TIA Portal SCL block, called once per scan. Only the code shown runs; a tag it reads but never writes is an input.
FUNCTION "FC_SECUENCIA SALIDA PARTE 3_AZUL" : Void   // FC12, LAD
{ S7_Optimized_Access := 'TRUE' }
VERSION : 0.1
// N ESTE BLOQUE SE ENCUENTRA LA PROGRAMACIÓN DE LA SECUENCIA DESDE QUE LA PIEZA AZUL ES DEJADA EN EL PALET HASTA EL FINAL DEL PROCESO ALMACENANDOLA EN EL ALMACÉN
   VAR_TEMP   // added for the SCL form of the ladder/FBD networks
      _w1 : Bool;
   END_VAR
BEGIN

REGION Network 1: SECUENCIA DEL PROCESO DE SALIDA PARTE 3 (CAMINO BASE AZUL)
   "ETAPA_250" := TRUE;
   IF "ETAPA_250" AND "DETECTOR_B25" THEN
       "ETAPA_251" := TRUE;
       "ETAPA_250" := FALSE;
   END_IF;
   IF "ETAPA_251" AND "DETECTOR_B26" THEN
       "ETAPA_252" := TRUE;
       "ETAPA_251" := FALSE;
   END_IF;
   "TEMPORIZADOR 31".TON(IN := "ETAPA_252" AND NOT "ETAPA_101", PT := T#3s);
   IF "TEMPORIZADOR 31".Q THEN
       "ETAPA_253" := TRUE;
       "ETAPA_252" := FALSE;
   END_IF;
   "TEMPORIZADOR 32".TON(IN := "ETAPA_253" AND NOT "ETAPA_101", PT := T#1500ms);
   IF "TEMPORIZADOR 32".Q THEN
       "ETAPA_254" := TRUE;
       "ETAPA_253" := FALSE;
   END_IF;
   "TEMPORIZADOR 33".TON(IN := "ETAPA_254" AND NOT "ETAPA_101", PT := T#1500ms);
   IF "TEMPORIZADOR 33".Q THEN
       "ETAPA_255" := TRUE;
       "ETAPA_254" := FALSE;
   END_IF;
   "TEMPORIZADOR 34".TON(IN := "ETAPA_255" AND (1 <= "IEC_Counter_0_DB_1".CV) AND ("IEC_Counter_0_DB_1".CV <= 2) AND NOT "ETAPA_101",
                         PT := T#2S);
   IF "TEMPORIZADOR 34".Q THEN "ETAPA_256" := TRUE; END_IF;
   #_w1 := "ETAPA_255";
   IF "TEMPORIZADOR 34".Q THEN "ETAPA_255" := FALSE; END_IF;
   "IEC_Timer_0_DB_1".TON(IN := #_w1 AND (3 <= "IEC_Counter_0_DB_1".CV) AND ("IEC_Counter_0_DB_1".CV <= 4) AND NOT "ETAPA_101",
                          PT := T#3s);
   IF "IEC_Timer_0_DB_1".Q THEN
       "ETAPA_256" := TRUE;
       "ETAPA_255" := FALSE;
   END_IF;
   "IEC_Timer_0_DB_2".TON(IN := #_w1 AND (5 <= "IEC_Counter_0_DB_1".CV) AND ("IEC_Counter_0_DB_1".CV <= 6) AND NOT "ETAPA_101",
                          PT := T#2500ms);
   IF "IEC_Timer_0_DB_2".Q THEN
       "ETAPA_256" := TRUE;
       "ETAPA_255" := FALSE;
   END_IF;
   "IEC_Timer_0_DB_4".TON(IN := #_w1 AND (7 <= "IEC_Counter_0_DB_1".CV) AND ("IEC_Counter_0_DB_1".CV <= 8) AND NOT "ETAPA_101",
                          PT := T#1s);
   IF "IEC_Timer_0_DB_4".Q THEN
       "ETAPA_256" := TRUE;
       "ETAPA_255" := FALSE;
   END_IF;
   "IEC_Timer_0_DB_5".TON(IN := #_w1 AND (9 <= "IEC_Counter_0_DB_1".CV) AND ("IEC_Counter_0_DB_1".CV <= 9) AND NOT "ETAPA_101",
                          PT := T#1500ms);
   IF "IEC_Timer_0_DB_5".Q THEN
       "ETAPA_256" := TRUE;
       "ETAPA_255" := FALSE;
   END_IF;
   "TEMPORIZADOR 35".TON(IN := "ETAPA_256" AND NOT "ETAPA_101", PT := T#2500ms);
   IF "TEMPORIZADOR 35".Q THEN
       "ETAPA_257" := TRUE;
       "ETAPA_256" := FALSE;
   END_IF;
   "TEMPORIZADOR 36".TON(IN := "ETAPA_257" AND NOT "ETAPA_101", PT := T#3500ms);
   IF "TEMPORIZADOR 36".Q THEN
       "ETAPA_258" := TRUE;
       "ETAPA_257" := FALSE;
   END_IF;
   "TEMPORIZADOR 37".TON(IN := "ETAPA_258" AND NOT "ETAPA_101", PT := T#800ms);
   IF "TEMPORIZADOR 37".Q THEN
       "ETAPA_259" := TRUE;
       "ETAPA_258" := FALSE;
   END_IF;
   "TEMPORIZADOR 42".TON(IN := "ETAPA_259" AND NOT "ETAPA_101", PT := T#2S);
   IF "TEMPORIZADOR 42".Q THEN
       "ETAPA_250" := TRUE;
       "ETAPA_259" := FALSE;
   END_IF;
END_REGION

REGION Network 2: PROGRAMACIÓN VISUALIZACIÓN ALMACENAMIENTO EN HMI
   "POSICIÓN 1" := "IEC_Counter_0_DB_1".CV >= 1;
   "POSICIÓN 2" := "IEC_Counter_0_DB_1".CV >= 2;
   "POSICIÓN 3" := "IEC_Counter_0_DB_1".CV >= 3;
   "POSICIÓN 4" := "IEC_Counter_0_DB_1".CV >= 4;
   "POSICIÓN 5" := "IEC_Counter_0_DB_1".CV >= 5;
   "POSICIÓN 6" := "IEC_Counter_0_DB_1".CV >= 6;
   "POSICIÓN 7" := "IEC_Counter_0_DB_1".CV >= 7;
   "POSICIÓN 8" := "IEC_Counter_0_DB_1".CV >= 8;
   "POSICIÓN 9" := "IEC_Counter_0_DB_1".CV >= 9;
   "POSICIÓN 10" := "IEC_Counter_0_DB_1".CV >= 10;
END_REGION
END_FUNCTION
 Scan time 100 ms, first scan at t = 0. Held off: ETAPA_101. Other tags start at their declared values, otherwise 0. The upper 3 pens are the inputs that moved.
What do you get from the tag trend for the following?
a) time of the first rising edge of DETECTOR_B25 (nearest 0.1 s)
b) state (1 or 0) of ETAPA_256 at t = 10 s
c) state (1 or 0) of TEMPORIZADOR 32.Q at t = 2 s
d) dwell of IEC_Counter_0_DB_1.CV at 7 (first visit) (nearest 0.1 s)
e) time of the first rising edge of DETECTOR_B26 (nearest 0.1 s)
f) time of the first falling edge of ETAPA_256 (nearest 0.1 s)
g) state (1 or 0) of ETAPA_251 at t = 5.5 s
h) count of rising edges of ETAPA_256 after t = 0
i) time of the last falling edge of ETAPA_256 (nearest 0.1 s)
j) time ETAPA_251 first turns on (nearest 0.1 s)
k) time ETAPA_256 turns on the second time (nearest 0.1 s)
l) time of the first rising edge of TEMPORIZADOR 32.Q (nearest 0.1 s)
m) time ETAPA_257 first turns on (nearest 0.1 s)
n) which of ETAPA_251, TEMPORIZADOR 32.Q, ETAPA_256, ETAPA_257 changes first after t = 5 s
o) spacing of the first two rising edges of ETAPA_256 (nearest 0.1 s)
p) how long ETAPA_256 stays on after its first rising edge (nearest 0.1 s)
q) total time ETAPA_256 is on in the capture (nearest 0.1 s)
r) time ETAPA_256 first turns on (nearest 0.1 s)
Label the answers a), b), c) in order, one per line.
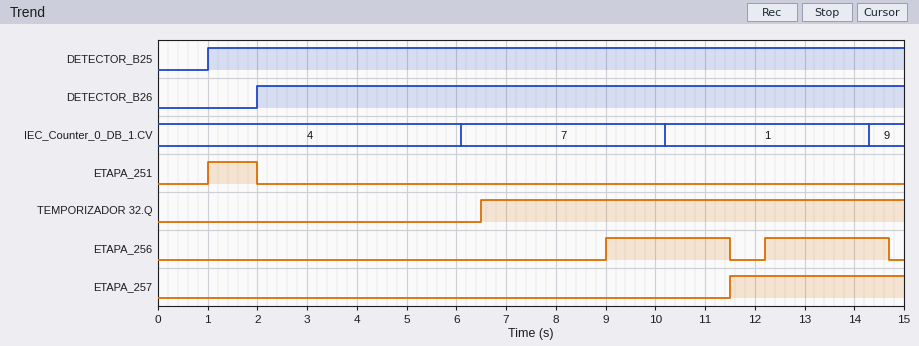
a) 1.0 s
b) 1
c) 0
d) 4.1 s
e) 2.0 s
f) 11.5 s
g) 0
h) 2
i) 14.7 s
j) 1.0 s
k) 12.2 s
l) 6.5 s
m) 11.5 s
n) TEMPORIZADOR 32.Q
o) 3.2 s
p) 2.5 s
q) 5.0 s
r) 9.0 s
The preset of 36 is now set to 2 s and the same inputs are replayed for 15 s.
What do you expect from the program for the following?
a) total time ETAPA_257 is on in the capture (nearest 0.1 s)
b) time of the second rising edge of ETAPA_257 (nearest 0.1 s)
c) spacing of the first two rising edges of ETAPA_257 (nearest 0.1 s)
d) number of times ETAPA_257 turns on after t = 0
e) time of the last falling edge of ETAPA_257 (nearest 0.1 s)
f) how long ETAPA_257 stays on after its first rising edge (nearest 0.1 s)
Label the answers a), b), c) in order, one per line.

a) 2.3 s
b) 14.7 s
c) 3.2 s
d) 2
e) 13.5 s
f) 2.0 s
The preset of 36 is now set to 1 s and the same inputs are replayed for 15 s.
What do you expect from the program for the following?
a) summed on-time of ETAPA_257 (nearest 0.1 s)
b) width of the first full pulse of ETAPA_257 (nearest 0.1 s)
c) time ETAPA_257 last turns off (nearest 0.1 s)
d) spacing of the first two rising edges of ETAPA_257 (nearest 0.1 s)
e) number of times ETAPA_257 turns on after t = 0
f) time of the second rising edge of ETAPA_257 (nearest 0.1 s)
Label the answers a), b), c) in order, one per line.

a) 1.3 s
b) 1.0 s
c) 12.5 s
d) 3.2 s
e) 2
f) 14.7 s
